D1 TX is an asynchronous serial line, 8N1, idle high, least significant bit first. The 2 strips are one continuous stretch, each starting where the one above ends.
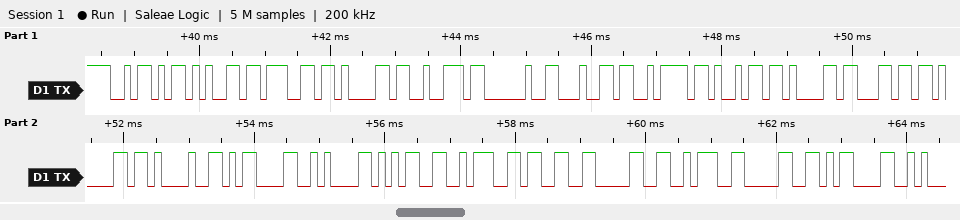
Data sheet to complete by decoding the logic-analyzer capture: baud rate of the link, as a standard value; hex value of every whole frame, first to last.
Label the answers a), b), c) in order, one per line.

a) 9600 baud
b) 0x5A 0x65 0x67 0x61 0x72 0x20 0x64 0x7A 0x69 0x61 0x6C 0x61 0x21 0x0D 0x0A 0x35 0x3A 0x33 0x30 0x3A 0x30 0x0D
